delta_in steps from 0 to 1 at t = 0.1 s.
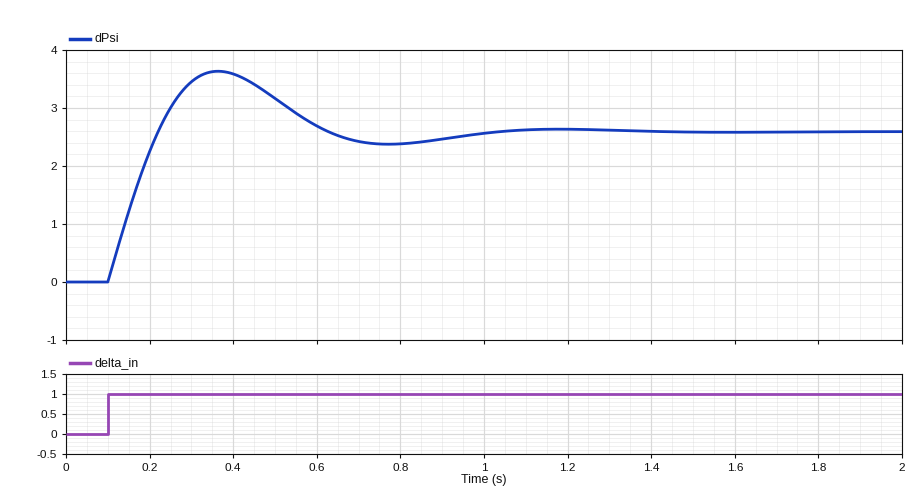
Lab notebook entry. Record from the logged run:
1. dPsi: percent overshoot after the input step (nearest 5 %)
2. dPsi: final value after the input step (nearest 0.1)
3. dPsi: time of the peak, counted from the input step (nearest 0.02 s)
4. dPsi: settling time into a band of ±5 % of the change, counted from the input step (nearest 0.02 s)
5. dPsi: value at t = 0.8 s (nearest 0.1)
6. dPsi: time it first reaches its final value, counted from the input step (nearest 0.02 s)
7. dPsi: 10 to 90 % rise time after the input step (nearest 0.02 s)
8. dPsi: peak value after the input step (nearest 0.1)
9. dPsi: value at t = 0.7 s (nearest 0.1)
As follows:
40 %
2.6
0.26 s
0.80 s
2.4
0.12 s
0.10 s
3.6
2.4
